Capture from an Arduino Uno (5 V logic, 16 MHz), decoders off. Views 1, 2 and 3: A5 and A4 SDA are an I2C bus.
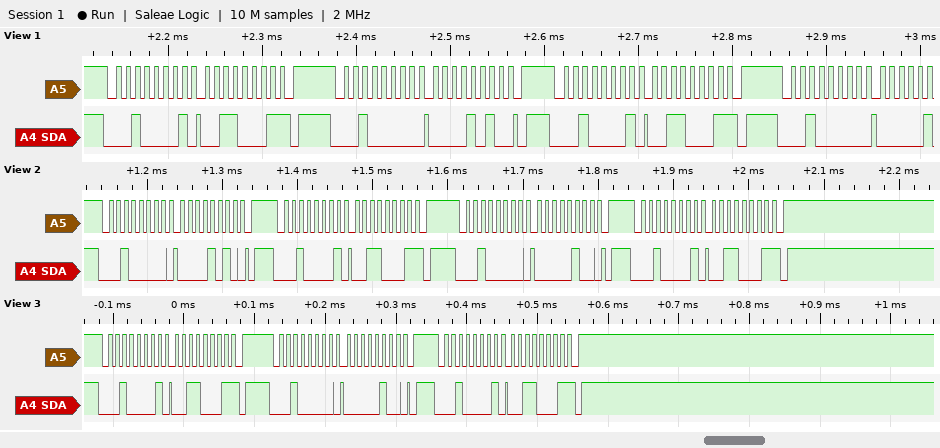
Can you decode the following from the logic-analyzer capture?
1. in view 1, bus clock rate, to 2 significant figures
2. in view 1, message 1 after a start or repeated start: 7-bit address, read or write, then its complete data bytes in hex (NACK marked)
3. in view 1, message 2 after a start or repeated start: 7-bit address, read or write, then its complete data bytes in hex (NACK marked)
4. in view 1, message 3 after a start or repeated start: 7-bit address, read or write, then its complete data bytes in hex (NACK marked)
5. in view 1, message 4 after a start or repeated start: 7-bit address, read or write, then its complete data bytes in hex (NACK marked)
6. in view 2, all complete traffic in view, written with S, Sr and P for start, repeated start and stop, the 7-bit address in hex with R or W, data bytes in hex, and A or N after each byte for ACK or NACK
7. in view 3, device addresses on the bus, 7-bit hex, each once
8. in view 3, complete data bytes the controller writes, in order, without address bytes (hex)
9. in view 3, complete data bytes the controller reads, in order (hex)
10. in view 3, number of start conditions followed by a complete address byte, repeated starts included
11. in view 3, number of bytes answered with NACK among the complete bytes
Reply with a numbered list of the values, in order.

1. 100 kHz
2. 0x10 read: 31 NACK
3. 0x10 write: 0A
4. 0x10 read: 31 NACK
5. 0x10 write
6. S 10W A 0A A P S 10R A 31 N P S 10W A 04 A P S 10R A 31 N P
7. 0x10
8. 04
9. 31 31
10. 3
11. 2
